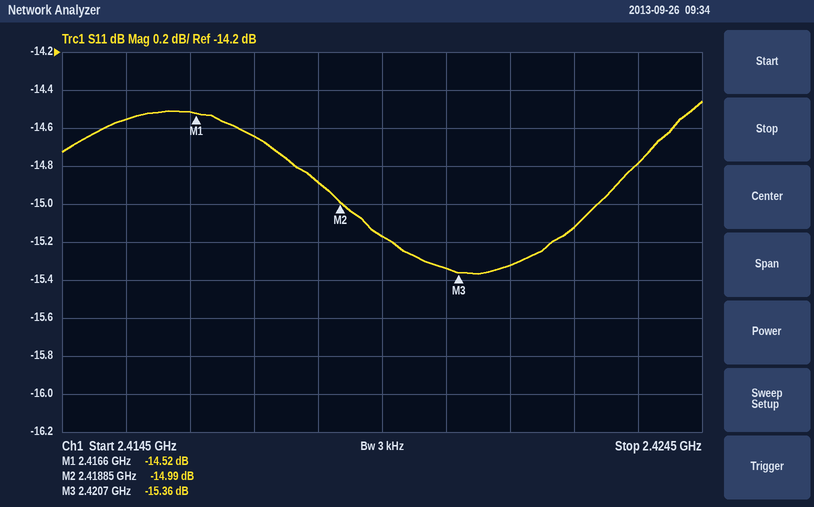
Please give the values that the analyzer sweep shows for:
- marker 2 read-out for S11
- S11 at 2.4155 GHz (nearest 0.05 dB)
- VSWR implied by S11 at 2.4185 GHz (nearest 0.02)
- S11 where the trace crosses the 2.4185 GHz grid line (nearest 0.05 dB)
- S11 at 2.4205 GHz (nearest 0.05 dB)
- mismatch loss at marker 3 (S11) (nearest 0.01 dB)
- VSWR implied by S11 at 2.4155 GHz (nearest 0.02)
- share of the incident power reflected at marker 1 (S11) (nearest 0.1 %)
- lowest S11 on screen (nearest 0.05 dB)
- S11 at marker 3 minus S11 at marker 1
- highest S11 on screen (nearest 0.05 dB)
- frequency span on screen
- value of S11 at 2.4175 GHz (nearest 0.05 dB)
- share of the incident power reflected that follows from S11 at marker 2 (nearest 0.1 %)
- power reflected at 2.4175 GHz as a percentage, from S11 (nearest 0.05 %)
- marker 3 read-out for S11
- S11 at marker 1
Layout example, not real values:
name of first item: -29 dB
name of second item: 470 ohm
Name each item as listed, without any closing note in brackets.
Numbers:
marker 2 read-out for S11: -14.99 dB
S11 at 2.4155 GHz: -14.55 dB
VSWR implied by S11 at 2.4185 GHz: 1.44
S11 where the trace crosses the 2.4185 GHz grid line: -14.90 dB
S11 at 2.4205 GHz: -15.35 dB
mismatch loss at marker 3 (S11): 0.13 dB
VSWR implied by S11 at 2.4155 GHz: 1.46
share of the incident power reflected at marker 1 (S11): 3.5 %
lowest S11 on screen: -15.35 dB
S11 at marker 3 minus S11 at marker 1: -0.84 dB
highest S11 on screen: -14.45 dB
frequency span on screen: 10 MHz
value of S11 at 2.4175 GHz: -14.65 dB
share of the incident power reflected that follows from S11 at marker 2: 3.2 %
power reflected at 2.4175 GHz as a percentage, from S11: 3.45 %
marker 3 read-out for S11: -15.36 dB
S11 at marker 1: -14.52 dB
